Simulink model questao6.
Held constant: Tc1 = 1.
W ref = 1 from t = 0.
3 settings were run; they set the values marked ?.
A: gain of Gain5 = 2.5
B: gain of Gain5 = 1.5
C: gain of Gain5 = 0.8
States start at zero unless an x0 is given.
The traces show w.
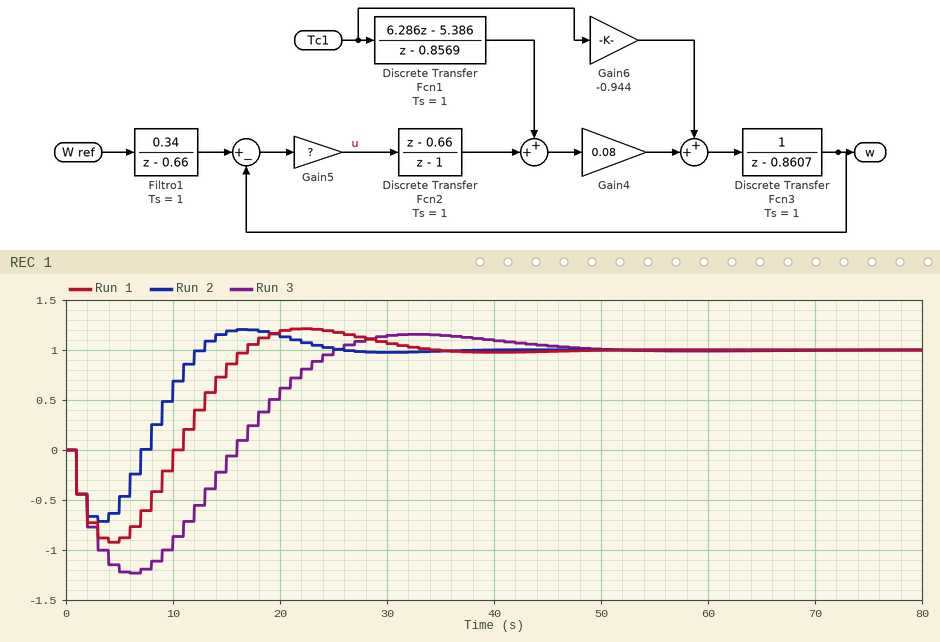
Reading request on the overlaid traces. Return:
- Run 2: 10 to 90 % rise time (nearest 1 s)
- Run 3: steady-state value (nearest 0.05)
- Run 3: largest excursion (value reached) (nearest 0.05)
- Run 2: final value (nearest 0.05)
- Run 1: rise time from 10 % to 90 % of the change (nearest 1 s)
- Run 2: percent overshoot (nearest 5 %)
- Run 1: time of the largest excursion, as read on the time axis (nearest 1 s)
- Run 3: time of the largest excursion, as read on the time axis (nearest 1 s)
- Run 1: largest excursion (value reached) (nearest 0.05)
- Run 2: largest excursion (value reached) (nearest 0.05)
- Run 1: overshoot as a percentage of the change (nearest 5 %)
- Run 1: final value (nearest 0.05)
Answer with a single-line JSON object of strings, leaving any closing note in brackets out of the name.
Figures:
{"Run 2: 10 to 90 % rise time": "4 s", "Run 3: steady-state value": "1.00", "Run 3: largest excursion (value reached)": "1.15", "Run 2: final value": "1.00", "Run 1: rise time from 10 % to 90 % of the change": "5 s", "Run 2: percent overshoot": "20 %", "Run 1: time of the largest excursion, as read on the time axis": "22 s", "Run 3: time of the largest excursion, as read on the time axis": "32 s", "Run 1: largest excursion (value reached)": "1.20", "Run 2: largest excursion (value reached)": "1.20", "Run 1: overshoot as a percentage of the change": "20 %", "Run 1: final value": "1.00"}
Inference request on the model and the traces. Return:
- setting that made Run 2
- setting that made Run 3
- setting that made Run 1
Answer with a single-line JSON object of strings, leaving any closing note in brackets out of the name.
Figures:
{"setting that made Run 2": "A", "setting that made Run 3": "C", "setting that made Run 1": "B"}
